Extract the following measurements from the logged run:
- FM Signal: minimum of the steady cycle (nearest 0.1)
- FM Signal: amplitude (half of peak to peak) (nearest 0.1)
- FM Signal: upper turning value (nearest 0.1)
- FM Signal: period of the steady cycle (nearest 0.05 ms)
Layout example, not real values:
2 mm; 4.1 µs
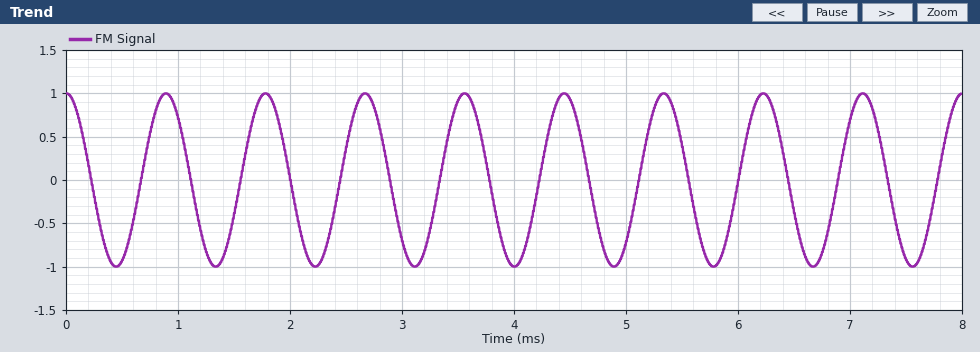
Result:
-1.0; 1.0; 1.0; 0.90 ms
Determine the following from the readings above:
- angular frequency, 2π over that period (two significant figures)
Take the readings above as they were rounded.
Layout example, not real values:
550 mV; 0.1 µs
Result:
7.0 rad/ms
